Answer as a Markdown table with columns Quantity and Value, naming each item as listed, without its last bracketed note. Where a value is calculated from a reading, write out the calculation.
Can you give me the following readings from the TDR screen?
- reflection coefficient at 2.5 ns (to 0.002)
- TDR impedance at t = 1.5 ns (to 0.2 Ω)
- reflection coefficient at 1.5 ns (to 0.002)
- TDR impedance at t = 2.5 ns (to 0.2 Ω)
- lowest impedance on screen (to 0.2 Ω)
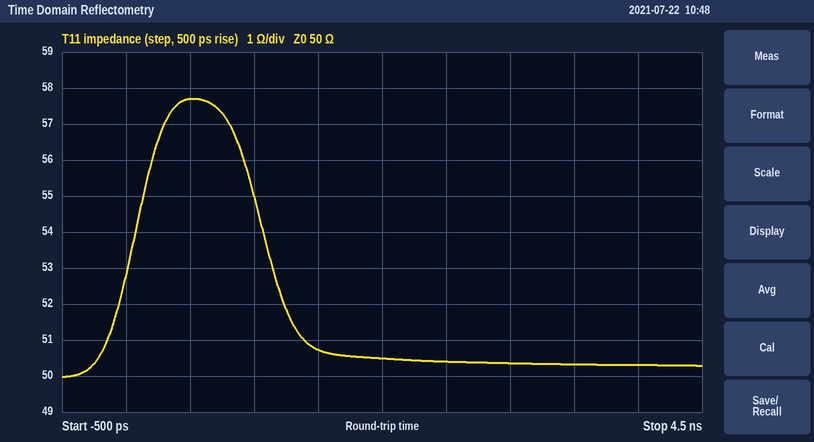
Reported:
| Quantity | Value |
|---|---|
| reflection coefficient at 2.5 ns | (50.4 − 50)/(50.4 + 50) ≈ +0.004 |
| TDR impedance at t = 1.5 ns | 50.8 Ω |
| reflection coefficient at 1.5 ns | (50.8 − 50)/(50.8 + 50) ≈ +0.008 |
| TDR impedance at t = 2.5 ns | 50.4 Ω |
| lowest impedance on screen | 50.0 Ω |
